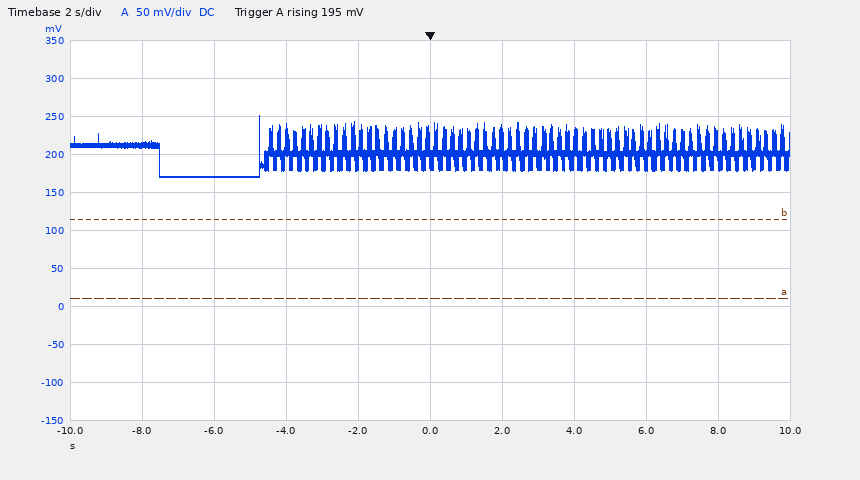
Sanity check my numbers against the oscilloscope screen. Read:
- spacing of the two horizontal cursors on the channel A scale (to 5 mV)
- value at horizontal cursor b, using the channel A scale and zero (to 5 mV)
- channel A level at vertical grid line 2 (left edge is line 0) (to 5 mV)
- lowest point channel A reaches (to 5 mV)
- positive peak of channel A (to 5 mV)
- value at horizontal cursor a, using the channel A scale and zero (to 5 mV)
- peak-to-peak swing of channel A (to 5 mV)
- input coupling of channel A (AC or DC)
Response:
105 mV
115 mV
170 mV
170 mV
250 mV
10 mV
80 mV
DC
